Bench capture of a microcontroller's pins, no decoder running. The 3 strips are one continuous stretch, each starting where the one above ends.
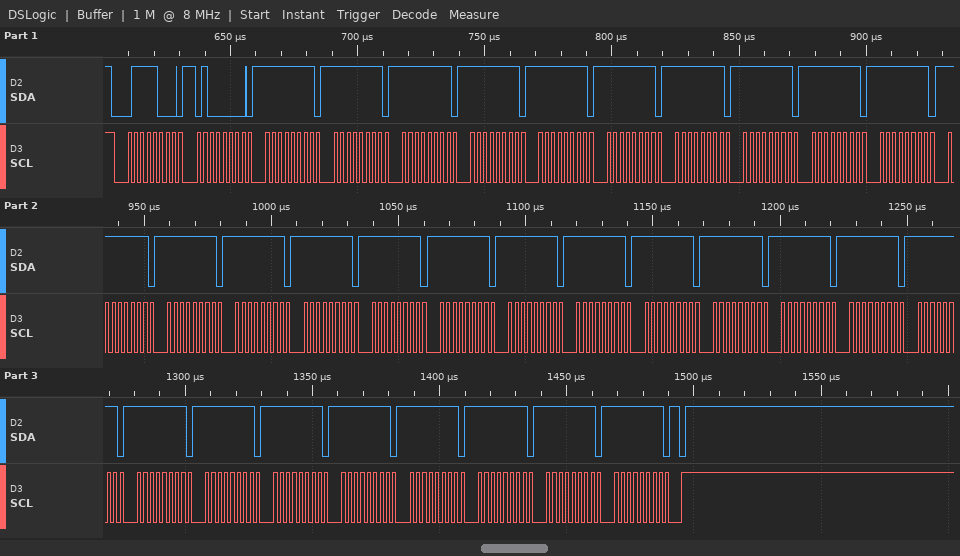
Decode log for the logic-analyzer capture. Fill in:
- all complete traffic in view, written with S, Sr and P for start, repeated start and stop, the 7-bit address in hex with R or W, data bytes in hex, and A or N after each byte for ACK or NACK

S 3CW A 40 A FF A FF A FF A FF A FF A FF A FF A FF A FF A FF A FF A FF A FF A FF A FF A FF A FF A FF A FF A FF A FF A FF A FF A FF A FF A FF A FF A FF A FF A FF A FF A P
